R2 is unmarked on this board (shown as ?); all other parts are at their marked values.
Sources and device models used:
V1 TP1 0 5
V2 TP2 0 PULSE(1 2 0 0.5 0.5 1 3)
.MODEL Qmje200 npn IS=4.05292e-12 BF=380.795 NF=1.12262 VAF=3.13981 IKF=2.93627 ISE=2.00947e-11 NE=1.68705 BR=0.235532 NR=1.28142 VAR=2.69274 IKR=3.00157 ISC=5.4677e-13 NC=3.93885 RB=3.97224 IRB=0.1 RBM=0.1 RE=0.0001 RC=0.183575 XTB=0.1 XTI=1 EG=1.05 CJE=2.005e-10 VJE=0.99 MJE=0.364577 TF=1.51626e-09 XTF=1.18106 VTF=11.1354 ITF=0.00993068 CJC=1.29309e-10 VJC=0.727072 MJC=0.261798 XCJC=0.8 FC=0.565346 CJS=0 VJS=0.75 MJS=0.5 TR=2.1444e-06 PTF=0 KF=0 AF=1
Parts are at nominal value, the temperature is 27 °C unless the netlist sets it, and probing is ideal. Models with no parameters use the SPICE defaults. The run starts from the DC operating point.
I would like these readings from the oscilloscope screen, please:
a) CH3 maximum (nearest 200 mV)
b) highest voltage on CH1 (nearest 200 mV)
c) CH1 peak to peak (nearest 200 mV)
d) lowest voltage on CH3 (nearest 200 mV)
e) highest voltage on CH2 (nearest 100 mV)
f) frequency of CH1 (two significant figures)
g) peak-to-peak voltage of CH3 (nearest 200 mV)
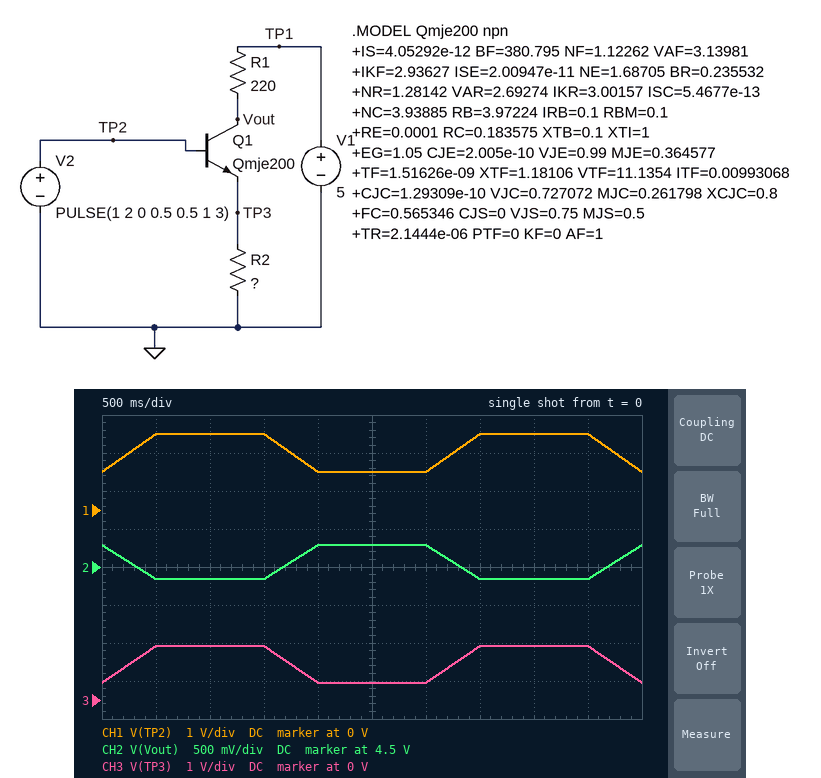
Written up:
1.4 V
2.0 V
1.0 V
400 mV
4.8 V
330 mHz
1.0 V
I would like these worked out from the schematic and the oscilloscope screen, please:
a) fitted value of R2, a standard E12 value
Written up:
470 Ω
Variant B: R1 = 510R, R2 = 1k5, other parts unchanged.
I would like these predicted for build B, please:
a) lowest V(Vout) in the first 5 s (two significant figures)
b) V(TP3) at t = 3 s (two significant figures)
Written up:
4.5 V
490 mV
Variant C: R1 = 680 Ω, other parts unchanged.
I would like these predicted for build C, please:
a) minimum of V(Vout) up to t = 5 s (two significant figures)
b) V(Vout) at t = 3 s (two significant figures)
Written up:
3.0 V
4.3 V
